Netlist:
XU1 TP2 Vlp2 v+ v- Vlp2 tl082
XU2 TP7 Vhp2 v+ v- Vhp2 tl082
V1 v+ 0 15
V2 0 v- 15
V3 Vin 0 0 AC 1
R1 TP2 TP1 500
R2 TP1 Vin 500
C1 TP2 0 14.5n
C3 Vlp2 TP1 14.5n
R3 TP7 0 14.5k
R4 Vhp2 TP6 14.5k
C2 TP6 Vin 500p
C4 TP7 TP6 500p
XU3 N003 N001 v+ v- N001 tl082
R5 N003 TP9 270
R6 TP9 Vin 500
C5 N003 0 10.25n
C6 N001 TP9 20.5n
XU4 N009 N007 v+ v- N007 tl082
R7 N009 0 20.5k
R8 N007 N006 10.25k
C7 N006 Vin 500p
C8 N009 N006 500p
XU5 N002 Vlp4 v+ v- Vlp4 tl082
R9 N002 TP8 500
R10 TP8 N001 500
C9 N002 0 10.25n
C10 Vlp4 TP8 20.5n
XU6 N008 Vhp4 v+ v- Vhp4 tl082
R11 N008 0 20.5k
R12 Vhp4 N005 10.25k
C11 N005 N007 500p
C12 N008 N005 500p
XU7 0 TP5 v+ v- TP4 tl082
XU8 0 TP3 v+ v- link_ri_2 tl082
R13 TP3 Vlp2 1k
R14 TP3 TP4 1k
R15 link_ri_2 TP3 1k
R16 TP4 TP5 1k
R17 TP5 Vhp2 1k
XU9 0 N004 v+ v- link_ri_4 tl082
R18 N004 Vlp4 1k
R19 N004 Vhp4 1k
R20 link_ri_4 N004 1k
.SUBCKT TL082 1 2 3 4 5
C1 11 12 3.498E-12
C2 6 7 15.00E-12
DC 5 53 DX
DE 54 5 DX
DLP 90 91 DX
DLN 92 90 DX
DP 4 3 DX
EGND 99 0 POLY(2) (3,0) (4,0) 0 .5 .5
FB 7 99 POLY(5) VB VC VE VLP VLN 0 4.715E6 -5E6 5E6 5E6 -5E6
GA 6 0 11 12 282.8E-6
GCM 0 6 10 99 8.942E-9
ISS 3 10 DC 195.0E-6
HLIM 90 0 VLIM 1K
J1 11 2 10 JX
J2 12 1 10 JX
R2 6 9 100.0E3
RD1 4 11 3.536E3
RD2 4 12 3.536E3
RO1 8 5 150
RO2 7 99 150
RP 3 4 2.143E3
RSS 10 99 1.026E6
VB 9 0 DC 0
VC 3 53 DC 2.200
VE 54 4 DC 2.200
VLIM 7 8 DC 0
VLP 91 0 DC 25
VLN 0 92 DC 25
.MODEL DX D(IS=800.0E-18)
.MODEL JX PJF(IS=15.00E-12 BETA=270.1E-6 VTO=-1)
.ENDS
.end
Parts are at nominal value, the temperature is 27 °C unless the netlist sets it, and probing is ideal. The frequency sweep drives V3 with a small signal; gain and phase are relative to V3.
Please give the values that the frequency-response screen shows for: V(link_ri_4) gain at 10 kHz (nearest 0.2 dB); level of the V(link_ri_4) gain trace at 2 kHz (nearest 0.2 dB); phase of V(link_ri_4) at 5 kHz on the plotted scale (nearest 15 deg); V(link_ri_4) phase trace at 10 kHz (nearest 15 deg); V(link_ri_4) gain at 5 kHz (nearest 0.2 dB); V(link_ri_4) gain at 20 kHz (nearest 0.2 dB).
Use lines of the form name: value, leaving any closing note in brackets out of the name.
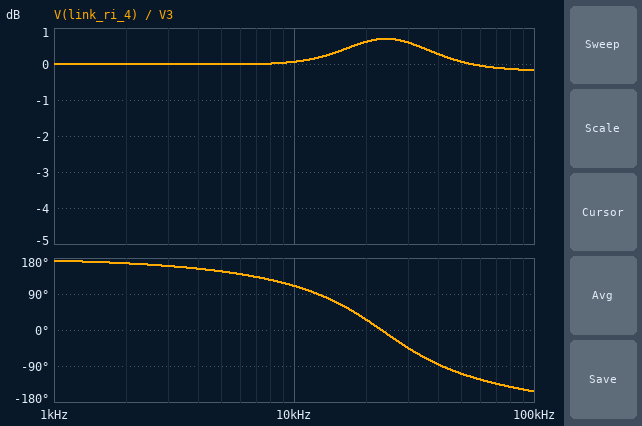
V(link_ri_4) gain at 10 kHz: 0 dB
level of the V(link_ri_4) gain trace at 2 kHz: 0 dB
phase of V(link_ri_4) at 5 kHz on the plotted scale: 150 deg
V(link_ri_4) phase trace at 10 kHz: 105 deg
V(link_ri_4) gain at 5 kHz: 0 dB
V(link_ri_4) gain at 20 kHz: 0.6 dB
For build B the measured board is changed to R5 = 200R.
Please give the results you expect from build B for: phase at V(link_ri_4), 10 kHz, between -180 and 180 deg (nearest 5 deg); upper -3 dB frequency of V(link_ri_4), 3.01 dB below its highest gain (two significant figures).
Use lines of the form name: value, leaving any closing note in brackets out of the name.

phase at V(link_ri_4), 10 kHz, between -180 and 180 deg: 115 deg
upper -3 dB frequency of V(link_ri_4), 3.01 dB below its highest gain: 970 kHz
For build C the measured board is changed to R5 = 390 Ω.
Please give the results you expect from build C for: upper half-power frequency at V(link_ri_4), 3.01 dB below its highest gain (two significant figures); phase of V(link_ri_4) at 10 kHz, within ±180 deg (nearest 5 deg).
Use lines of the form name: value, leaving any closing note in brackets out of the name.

upper half-power frequency at V(link_ri_4), 3.01 dB below its highest gain: 1.0 MHz
phase of V(link_ri_4) at 10 kHz, within ±180 deg: 105 deg
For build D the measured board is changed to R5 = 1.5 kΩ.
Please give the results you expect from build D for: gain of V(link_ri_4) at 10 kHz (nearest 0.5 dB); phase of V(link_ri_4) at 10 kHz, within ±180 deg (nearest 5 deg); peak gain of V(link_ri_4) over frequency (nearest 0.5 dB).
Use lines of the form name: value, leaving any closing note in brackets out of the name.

gain of V(link_ri_4) at 10 kHz: -2.5 dB
phase of V(link_ri_4) at 10 kHz, within ±180 deg: 70 deg
peak gain of V(link_ri_4) over frequency: 0 dB
